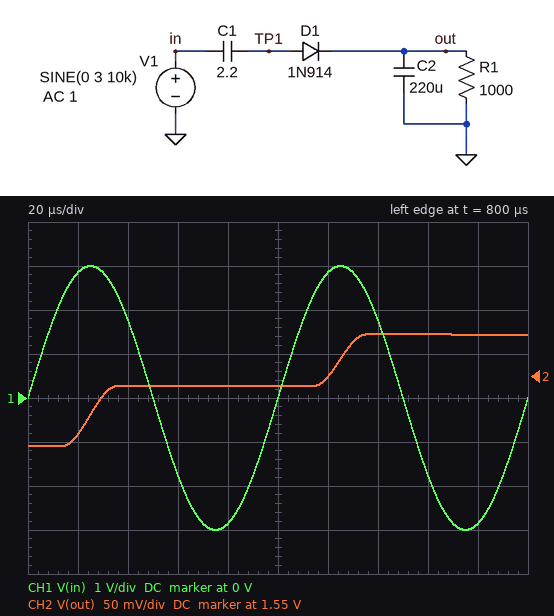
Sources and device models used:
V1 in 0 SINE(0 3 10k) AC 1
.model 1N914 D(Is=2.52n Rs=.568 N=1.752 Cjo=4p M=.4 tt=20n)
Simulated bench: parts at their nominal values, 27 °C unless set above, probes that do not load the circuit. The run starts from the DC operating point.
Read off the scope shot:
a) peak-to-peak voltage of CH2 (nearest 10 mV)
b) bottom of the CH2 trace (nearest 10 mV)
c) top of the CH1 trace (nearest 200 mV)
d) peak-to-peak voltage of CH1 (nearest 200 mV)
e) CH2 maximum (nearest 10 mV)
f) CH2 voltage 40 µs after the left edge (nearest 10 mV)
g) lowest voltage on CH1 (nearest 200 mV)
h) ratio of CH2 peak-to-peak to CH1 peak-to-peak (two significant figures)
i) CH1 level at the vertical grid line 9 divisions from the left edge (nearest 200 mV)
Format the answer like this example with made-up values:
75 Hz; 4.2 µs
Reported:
130 mV; 1.47 V; 3.0 V; 6.0 V; 1.60 V; 1.54 V; -3.0 V; 0.021; -2.8 V
